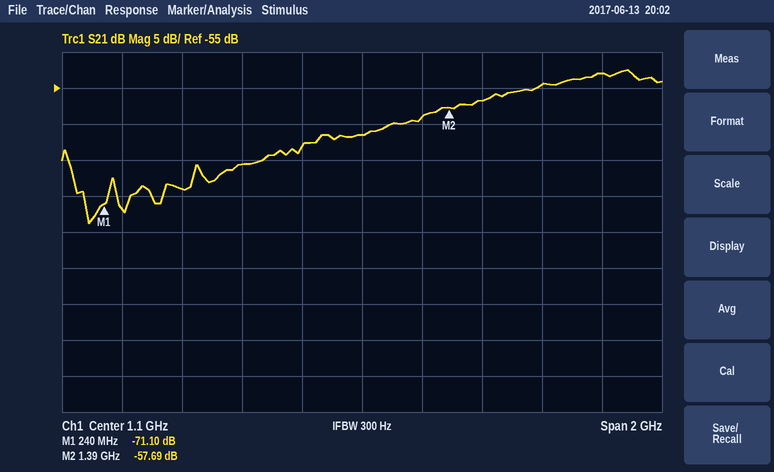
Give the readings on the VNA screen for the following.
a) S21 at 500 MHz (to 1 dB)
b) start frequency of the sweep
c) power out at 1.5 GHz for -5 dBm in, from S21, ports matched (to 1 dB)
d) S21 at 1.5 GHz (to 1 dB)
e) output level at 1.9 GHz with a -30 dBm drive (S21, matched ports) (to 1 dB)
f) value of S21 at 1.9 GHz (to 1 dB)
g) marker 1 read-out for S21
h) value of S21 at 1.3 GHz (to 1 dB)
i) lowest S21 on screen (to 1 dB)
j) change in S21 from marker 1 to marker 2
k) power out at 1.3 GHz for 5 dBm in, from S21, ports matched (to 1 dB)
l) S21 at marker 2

-69 dB
100 MHz
-62 dBm
-57 dB
-83 dBm
-53 dB
-71.10 dB
-59 dB
-74 dB
13.41 dB
-54 dBm
-57.69 dB
